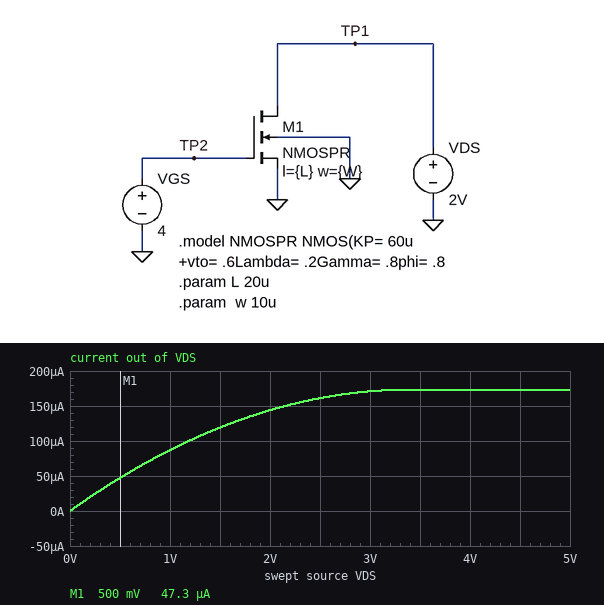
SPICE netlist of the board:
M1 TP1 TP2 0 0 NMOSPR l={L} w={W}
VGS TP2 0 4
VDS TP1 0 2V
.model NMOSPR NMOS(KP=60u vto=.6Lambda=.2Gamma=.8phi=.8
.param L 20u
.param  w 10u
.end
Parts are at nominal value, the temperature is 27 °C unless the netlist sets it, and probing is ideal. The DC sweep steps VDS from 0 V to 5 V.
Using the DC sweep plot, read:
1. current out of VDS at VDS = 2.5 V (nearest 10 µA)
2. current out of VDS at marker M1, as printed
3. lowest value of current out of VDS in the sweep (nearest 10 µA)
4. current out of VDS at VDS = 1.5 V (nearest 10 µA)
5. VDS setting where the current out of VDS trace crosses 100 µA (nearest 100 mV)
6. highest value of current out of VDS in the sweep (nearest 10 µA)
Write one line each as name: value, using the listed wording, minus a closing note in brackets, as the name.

current out of VDS at VDS = 2.5 V: 160 µA
current out of VDS at marker M1, as printed: 47.3 µA
lowest value of current out of VDS in the sweep: 0 A
current out of VDS at VDS = 1.5 V: 120 µA
VDS setting where the current out of VDS trace crosses 100 µA: 1.2 V
highest value of current out of VDS in the sweep: 170 µA
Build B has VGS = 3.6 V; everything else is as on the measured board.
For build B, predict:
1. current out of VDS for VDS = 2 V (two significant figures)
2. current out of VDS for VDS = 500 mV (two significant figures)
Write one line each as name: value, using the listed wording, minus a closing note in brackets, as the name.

current out of VDS for VDS = 2 V: 120 µA
current out of VDS for VDS = 500 mV: 41 µA
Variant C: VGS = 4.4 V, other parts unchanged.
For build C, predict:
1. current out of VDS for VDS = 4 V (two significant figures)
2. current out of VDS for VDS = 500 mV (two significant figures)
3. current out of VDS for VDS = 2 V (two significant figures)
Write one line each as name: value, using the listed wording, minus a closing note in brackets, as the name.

current out of VDS for VDS = 4 V: 220 µA
current out of VDS for VDS = 500 mV: 53 µA
current out of VDS for VDS = 2 V: 170 µA
